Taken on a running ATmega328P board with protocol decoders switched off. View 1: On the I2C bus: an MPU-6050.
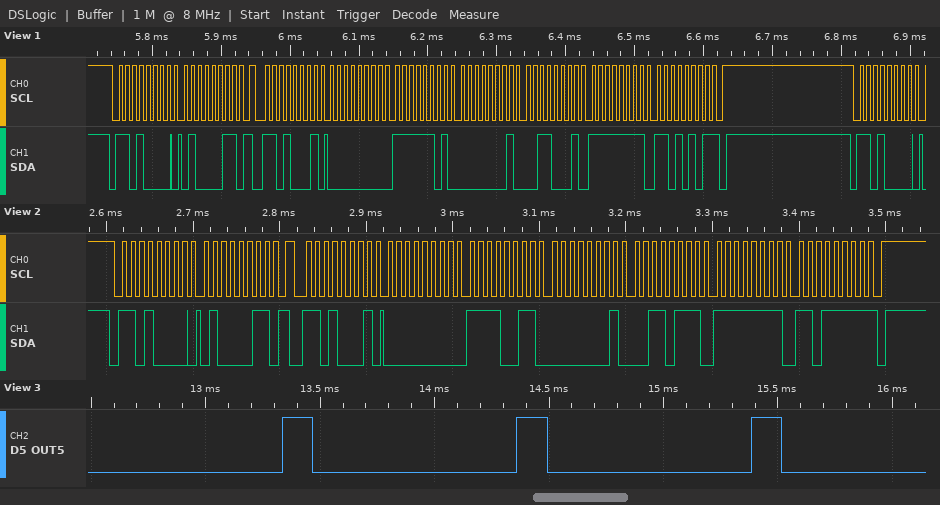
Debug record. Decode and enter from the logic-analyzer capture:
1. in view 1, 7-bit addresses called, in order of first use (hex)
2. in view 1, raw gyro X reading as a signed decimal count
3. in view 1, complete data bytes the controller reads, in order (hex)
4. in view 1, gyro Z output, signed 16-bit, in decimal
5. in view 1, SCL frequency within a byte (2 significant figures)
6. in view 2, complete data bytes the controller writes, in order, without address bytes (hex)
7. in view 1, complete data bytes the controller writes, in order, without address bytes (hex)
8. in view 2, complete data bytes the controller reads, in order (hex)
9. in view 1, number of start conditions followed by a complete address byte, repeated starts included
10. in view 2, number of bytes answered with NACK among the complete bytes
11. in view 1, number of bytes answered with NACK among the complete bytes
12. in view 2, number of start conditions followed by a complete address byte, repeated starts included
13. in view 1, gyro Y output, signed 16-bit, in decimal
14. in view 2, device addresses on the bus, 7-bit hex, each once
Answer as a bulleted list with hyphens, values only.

- 0x68
- 253
- 00 FD 01 31 FF D5
- -43
- 100 kHz
- 43
- 43
- 00 F3 01 37 FF DF
- 3
- 1
- 1
- 2
- 305
- 0x68
